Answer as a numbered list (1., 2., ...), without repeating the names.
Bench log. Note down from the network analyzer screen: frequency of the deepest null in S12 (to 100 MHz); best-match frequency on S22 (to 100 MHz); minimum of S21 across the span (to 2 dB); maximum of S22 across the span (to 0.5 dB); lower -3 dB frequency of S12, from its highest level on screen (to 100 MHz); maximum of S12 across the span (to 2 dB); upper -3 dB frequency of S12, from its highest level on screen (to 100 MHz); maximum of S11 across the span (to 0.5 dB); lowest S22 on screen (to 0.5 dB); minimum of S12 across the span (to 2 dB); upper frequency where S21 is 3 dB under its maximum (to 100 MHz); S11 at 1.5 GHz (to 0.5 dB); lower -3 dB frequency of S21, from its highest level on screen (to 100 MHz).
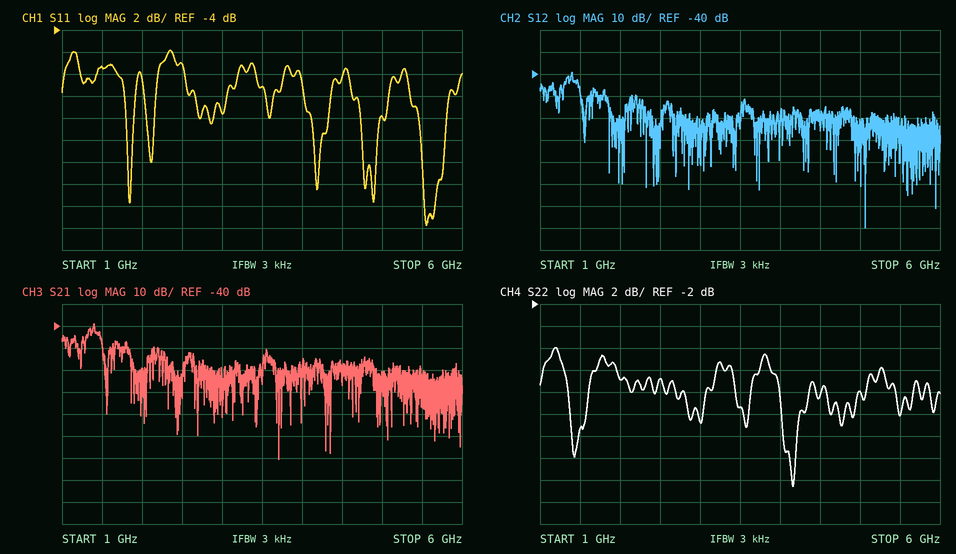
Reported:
1. 5.1 GHz
2. 4.2 GHz
3. -100 dB
4. -6.0 dB
5. 1.4 GHz
6. -40 dB
7. 1.4 GHz
8. -6.0 dB
9. -18.5 dB
10. -110 dB
11. 1.4 GHz
12. -7.5 dB
13. 1.4 GHz
